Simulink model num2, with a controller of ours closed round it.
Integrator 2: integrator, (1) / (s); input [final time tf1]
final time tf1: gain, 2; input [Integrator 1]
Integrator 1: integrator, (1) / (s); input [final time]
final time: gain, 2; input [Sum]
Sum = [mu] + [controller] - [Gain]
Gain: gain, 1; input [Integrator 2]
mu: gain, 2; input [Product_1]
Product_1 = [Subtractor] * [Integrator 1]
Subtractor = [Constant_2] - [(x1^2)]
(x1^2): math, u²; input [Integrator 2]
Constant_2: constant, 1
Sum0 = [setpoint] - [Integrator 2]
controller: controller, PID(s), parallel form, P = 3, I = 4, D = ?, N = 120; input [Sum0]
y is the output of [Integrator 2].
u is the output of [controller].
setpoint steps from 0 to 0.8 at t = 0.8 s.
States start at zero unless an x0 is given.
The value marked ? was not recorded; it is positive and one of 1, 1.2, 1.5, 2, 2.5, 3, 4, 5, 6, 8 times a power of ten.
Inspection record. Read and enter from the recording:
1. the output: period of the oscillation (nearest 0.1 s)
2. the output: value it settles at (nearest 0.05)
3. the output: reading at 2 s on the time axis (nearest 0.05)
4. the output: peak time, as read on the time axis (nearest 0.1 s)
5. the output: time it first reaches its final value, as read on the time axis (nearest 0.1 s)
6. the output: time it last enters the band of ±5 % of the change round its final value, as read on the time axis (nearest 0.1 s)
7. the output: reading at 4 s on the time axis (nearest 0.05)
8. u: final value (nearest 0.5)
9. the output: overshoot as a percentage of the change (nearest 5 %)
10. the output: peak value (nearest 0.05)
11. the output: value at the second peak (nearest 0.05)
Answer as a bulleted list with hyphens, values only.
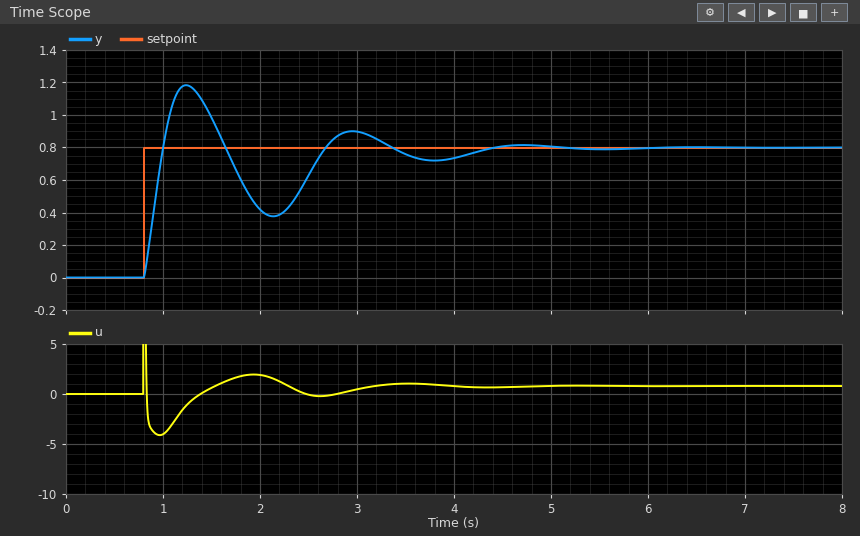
- 1.7 s
- 0.80
- 0.40
- 1.2 s
- 1.0 s
- 4.2 s
- 0.75
- 1.0
- 50 %
- 1.20
- 0.90
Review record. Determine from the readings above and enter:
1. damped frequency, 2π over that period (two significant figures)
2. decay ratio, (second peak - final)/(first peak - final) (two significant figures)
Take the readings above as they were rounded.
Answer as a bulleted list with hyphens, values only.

- 3.7 rad/s
- 0.25
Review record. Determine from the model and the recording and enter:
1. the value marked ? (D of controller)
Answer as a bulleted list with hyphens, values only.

- 1.2
